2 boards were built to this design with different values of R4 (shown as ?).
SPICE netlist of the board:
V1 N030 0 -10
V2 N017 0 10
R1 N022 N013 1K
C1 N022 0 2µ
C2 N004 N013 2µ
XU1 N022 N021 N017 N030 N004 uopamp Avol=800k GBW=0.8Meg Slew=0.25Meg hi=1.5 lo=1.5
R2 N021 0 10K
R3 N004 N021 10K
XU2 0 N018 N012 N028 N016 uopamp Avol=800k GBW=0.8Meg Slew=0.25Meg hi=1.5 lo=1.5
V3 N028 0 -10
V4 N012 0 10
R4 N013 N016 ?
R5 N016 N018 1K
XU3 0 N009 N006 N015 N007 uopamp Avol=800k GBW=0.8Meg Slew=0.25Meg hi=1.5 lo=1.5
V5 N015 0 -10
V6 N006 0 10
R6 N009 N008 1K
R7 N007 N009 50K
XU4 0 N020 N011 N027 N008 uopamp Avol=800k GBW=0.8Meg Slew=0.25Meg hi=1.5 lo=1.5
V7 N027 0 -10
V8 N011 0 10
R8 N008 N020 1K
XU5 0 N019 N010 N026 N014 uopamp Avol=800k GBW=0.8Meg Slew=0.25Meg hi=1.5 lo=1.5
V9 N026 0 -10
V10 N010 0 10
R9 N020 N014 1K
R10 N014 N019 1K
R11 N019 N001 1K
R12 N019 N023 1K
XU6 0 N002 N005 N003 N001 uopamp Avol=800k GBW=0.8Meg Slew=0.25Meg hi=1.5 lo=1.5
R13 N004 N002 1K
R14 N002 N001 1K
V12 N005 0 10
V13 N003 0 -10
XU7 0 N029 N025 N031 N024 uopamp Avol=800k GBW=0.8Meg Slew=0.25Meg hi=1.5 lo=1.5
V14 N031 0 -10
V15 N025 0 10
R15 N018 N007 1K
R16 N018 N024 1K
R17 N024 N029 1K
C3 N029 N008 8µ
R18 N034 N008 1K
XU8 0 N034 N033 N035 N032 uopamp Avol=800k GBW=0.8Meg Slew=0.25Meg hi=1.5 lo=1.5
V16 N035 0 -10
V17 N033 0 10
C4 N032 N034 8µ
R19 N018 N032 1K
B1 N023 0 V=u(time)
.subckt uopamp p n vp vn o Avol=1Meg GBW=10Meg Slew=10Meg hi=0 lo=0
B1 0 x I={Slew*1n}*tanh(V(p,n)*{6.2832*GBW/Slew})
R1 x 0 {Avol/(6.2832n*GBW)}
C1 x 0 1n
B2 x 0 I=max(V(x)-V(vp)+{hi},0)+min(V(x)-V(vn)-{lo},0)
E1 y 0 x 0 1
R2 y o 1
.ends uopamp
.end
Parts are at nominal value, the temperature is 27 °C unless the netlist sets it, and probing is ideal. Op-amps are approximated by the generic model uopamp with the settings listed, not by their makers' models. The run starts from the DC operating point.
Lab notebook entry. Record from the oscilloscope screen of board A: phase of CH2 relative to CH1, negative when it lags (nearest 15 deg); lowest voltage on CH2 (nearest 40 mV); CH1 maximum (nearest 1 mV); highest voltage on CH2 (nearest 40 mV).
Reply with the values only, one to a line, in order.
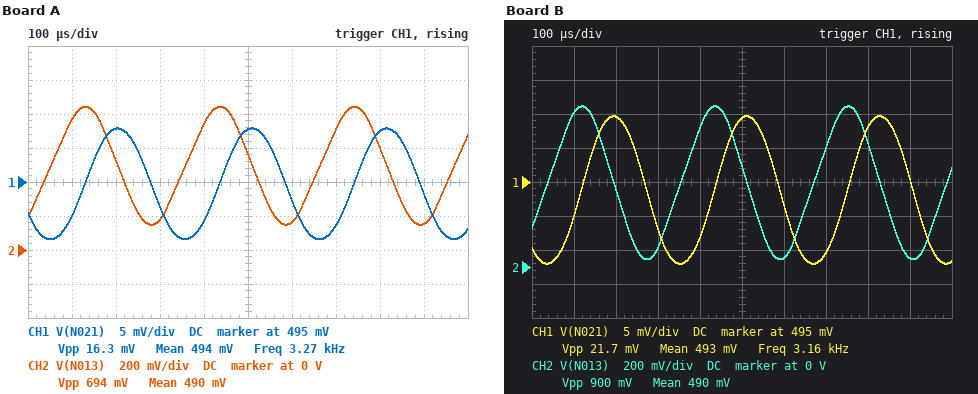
90 deg
160 mV
503 mV
840 mV
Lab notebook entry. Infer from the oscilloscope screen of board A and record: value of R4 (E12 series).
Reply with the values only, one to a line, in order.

680 Ω
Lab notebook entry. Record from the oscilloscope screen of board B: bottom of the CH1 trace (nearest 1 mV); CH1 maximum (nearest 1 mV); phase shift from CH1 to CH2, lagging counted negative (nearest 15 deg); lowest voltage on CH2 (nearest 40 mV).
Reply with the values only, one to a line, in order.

483 mV
505 mV
90 deg
40 mV
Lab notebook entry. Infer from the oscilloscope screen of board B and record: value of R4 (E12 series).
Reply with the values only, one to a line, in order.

560 Ω
